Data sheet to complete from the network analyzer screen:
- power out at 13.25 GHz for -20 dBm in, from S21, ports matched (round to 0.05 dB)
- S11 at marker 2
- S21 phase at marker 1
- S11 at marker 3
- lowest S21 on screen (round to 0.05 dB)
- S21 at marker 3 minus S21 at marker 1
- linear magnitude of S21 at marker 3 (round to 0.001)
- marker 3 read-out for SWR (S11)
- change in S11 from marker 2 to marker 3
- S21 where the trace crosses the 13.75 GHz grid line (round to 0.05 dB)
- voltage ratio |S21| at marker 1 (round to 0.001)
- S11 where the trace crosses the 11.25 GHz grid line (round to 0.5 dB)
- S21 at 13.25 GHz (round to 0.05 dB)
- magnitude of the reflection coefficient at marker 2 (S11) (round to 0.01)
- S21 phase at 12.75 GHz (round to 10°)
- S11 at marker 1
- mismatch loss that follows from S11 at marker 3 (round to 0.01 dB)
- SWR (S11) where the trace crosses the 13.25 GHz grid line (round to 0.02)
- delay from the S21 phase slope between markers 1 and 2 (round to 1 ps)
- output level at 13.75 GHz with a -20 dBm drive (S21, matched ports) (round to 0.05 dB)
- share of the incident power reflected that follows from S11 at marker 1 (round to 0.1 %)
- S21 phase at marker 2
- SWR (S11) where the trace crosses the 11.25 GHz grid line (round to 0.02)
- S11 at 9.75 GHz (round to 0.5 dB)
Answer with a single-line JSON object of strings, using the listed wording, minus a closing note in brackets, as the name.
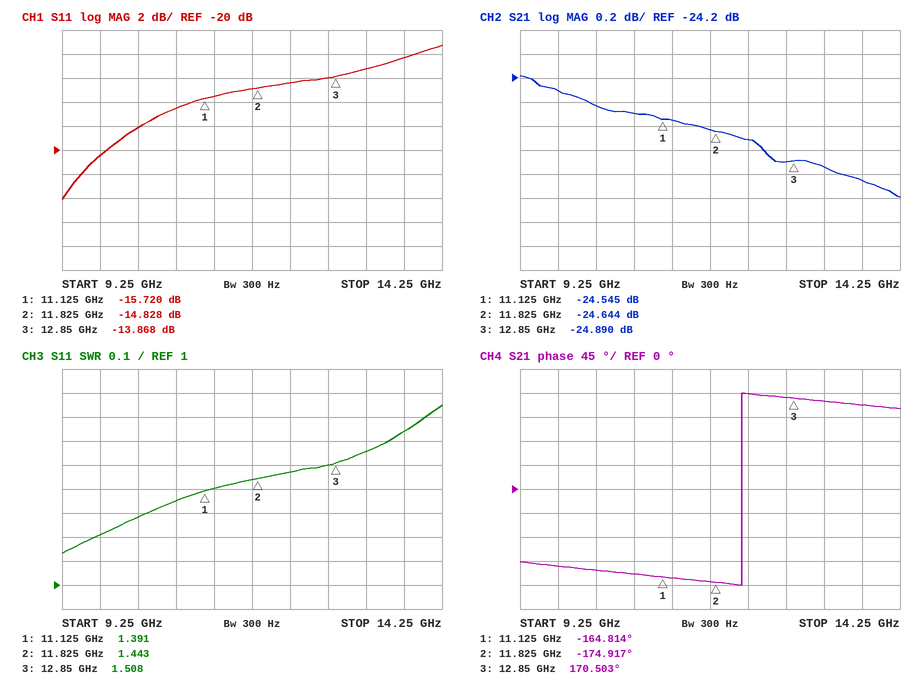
{"power out at 13.25 GHz for -20 dBm in, from S21, ports matched": "-44.95 dBm", "S11 at marker 2": "-14.828 dB", "S21 phase at marker 1": "-164.814°", "S11 at marker 3": "-13.868 dB", "lowest S21 on screen": "-25.20 dB", "S21 at marker 3 minus S21 at marker 1": "-0.345 dB", "linear magnitude of S21 at marker 3": "0.057", "marker 3 read-out for SWR": "1.508", "change in S11 from marker 2 to marker 3": "0.960 dB", "S21 where the trace crosses the 13.75 GHz grid line": "-25.05 dB", "voltage ratio |S21| at marker 1": "0.059", "S11 where the trace crosses the 11.25 GHz grid line": "-15.5 dB", "S21 at 13.25 GHz": "-24.95 dB", "magnitude of the reflection coefficient at marker 2 (S11)": "0.18", "S21 phase at 12.75 GHz": "170°", "S11 at marker 1": "-15.720 dB", "mismatch loss that follows from S11 at marker 3": "0.18 dB", "SWR (S11) where the trace crosses the 13.25 GHz grid line": "1.56", "delay from the S21 phase slope between markers 1 and 2": "40 ps", "output level at 13.75 GHz with a -20 dBm drive (S21, matched ports)": "-45.05 dBm", "share of the incident power reflected that follows from S11 at marker 1": "2.7 %", "S21 phase at marker 2": "-174.917°", "SWR (S11) where the trace crosses the 11.25 GHz grid line": "1.40", "S11 at 9.75 GHz": "-20.5 dB"}
